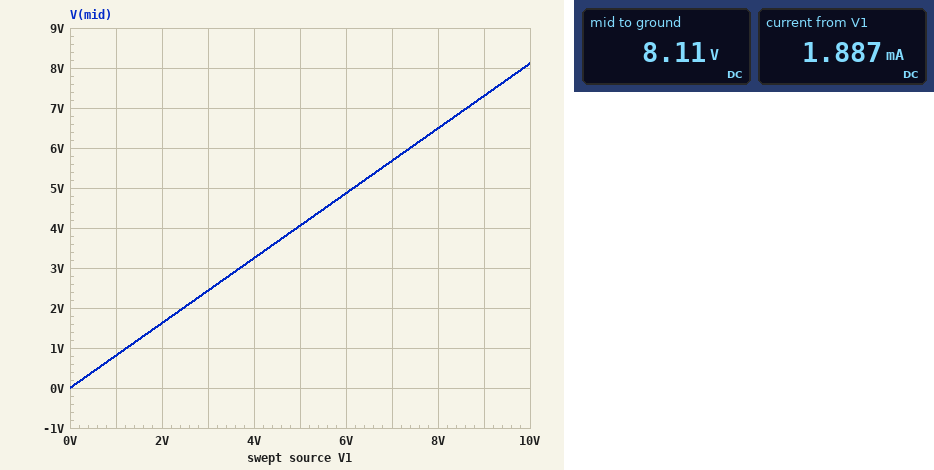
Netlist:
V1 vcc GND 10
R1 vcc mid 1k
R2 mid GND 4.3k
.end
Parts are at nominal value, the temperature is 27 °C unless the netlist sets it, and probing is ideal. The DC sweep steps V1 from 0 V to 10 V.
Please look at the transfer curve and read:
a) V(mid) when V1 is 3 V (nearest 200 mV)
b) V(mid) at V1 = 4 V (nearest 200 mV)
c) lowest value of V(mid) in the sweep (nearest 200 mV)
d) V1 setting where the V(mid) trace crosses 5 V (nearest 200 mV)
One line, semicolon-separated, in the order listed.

2.4 V; 3.2 V; 0 V; 6.2 V
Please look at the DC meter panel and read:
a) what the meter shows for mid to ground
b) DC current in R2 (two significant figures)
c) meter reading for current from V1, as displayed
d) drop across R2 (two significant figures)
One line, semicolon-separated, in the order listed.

8.11 V; 1.9 mA; 1.887 mA; 8.1 V
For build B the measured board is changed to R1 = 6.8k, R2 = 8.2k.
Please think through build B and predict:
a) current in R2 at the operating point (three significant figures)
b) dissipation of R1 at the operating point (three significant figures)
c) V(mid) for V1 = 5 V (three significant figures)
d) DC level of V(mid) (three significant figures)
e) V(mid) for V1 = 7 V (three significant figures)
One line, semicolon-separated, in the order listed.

667 µA; 3.02 mW; 2.73 V; 5.47 V; 3.83 V
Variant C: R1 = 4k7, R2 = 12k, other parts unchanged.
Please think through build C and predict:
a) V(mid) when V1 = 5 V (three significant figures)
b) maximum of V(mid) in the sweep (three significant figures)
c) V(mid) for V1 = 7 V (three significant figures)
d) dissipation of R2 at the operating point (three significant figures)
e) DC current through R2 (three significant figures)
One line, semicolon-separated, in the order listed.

3.59 V; 7.19 V; 5.03 V; 4.30 mW; 599 µA
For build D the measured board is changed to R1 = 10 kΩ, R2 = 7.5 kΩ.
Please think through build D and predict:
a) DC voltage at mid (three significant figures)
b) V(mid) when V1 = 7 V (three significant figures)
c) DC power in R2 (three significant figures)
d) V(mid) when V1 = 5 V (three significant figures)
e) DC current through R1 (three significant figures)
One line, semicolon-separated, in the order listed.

4.29 V; 3.00 V; 2.45 mW; 2.14 V; 571 µA
